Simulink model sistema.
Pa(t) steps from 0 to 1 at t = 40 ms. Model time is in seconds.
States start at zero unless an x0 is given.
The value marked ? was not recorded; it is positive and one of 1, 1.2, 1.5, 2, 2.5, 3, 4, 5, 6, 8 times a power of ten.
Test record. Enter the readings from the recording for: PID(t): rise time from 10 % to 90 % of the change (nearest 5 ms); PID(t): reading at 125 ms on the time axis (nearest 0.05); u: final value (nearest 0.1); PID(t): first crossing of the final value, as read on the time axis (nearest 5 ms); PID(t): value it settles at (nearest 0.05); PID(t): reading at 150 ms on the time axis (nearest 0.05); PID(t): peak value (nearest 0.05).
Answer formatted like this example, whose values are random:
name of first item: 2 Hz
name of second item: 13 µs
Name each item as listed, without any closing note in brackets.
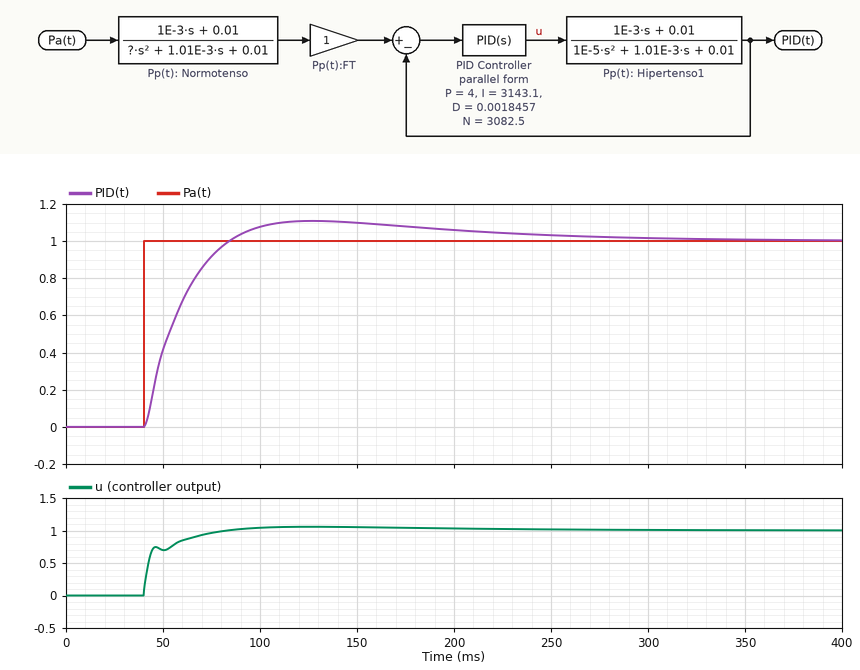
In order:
PID(t): rise time from 10 % to 90 % of the change: 30 ms
PID(t): reading at 125 ms on the time axis: 1.10
u: final value: 1.0
PID(t): first crossing of the final value, as read on the time axis: 85 ms
PID(t): value it settles at: 1.00
PID(t): reading at 150 ms on the time axis: 1.10
PID(t): peak value: 1.10
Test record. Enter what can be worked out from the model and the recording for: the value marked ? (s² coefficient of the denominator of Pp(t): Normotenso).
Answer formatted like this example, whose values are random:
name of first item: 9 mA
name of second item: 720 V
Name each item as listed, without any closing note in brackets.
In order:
the value marked ? (s² coefficient of the denominator of Pp(t): Normotenso): 2e-05
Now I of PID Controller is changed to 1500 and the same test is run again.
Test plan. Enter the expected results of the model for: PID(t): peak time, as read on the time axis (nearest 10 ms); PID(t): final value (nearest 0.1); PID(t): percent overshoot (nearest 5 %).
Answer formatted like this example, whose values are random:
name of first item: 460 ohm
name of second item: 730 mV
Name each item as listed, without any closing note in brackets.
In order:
PID(t): peak time, as read on the time axis: 130 ms
PID(t): final value: 1.0
PID(t): percent overshoot: 10 %
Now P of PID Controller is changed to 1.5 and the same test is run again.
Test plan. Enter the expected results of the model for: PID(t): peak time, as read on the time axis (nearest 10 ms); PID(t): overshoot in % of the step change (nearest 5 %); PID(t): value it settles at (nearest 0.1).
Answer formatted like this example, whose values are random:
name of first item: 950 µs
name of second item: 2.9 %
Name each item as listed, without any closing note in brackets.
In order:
PID(t): peak time, as read on the time axis: 130 ms
PID(t): overshoot in % of the step change: 10 %
PID(t): value it settles at: 1.0
